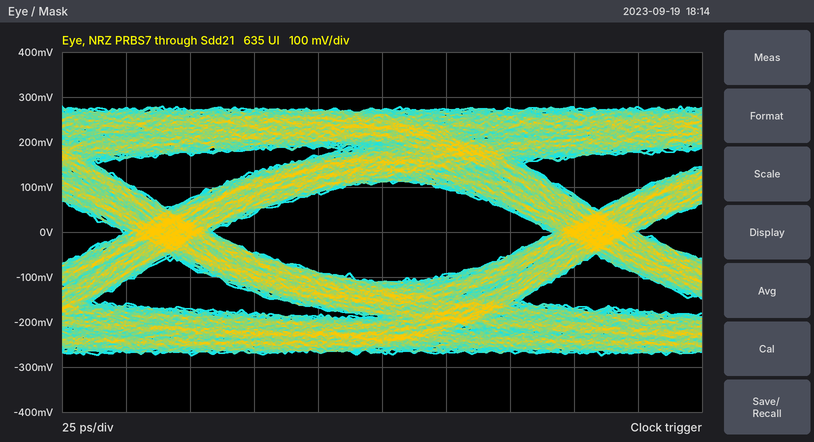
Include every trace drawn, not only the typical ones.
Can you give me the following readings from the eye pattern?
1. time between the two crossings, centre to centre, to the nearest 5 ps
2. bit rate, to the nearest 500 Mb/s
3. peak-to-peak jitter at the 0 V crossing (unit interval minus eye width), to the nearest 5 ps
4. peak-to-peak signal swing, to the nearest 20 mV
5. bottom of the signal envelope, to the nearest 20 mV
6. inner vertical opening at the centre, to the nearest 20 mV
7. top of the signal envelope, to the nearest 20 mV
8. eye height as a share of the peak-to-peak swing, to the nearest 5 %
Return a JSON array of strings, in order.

["165 ps", "6.0 Gb/s", "35 ps", "560 mV", "-280 mV", "220 mV", "280 mV", "40 %"]
